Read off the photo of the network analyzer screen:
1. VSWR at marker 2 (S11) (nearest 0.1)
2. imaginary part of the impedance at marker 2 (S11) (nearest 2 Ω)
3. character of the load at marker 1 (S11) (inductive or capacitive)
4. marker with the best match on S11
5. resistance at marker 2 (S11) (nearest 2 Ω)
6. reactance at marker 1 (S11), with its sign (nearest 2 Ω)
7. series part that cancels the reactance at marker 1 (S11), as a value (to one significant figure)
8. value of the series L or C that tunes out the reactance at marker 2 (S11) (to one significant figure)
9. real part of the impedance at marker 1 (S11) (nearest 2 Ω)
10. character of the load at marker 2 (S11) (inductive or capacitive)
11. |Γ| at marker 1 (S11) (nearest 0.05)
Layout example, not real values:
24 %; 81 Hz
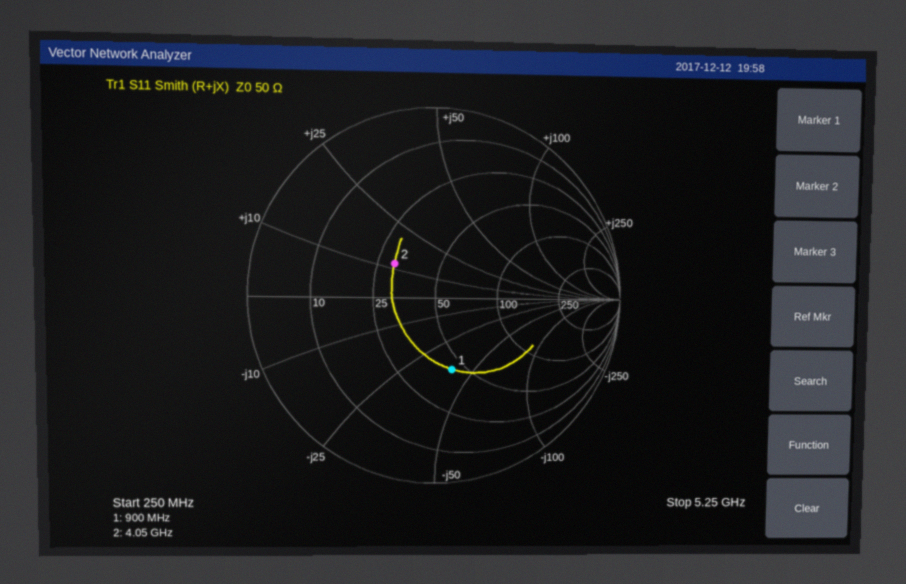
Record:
1.8; +12 Ω; capacitive; marker 2; 30 Ω; -40 Ω; 7 nH; 3 pF; 44 Ω; inductive; 0.40
